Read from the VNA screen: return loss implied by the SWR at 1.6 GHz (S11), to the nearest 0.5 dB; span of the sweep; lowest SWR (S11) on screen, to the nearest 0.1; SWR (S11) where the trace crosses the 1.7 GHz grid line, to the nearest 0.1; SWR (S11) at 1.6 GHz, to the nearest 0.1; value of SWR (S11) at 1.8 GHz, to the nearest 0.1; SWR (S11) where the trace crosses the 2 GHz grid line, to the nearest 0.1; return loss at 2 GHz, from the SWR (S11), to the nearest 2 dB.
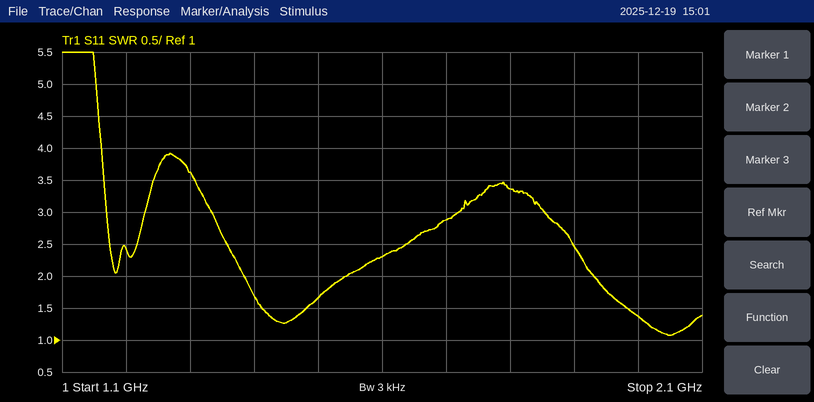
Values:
8.0 dB
1 GHz
1.1
2.9
2.3
3.4
1.4
16 dB
